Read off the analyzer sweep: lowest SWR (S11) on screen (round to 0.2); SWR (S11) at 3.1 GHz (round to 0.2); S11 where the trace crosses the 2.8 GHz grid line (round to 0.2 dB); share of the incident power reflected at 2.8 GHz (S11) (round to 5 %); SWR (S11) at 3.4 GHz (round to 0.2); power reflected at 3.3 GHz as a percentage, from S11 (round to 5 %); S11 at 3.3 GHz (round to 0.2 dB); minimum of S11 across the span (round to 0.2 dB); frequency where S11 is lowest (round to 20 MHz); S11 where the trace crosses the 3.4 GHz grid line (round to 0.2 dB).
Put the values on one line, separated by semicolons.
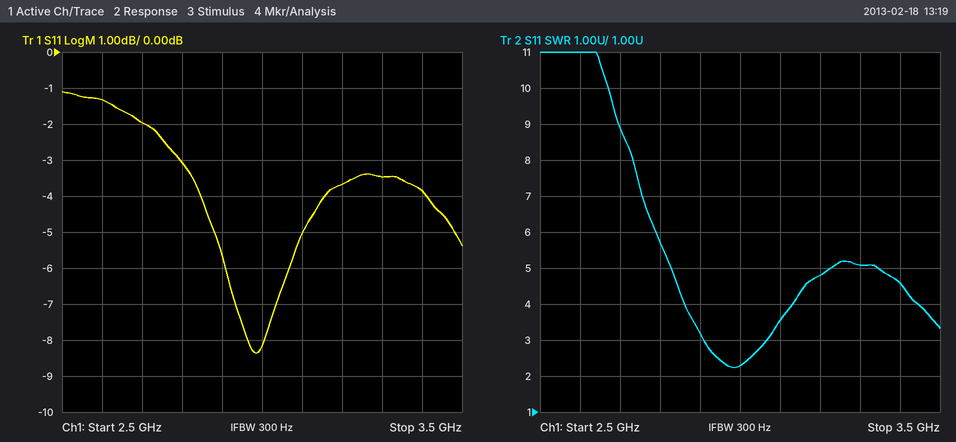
2.2; 3.6; -3.0 dB; 50 %; 4.6; 45 %; -3.4 dB; -8.4 dB; 2.98 GHz; -3.8 dB
